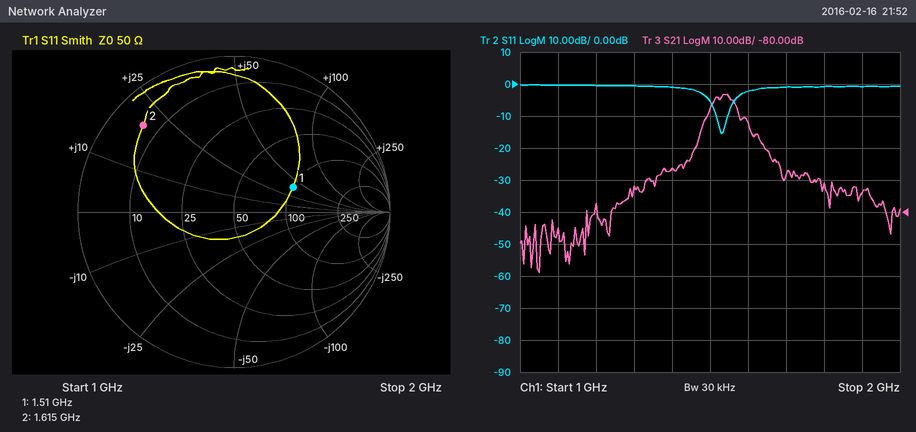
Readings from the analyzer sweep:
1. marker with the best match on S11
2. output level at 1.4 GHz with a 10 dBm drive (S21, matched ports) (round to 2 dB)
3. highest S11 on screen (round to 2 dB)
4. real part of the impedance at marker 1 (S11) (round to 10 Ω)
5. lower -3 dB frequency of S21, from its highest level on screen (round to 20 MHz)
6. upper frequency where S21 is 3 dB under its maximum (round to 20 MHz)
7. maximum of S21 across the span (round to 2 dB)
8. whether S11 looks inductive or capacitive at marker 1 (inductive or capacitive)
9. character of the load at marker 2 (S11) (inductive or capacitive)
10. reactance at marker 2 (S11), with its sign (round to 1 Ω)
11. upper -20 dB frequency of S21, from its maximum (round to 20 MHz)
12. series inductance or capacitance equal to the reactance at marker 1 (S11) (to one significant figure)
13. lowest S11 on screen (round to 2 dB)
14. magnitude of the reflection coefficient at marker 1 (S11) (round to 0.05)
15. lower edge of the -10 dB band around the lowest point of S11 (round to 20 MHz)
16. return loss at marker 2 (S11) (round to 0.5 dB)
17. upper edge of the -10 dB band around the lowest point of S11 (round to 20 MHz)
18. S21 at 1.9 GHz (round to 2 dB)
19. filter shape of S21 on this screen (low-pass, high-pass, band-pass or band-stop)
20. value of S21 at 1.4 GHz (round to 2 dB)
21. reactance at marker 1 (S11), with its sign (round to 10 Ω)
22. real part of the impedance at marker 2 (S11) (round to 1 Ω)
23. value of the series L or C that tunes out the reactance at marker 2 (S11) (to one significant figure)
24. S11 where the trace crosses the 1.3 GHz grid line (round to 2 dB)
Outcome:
marker 1
-56 dBm
0 dB
100 Ω
1.50 GHz
1.56 GHz
-44 dB
inductive
inductive
+20 Ω
1.66 GHz
4 nH
-16 dB
0.40
1.52 GHz
2.0 dB
1.54 GHz
-74 dB
band-pass
-66 dB
+40 Ω
6 Ω
5 pF
0 dB
